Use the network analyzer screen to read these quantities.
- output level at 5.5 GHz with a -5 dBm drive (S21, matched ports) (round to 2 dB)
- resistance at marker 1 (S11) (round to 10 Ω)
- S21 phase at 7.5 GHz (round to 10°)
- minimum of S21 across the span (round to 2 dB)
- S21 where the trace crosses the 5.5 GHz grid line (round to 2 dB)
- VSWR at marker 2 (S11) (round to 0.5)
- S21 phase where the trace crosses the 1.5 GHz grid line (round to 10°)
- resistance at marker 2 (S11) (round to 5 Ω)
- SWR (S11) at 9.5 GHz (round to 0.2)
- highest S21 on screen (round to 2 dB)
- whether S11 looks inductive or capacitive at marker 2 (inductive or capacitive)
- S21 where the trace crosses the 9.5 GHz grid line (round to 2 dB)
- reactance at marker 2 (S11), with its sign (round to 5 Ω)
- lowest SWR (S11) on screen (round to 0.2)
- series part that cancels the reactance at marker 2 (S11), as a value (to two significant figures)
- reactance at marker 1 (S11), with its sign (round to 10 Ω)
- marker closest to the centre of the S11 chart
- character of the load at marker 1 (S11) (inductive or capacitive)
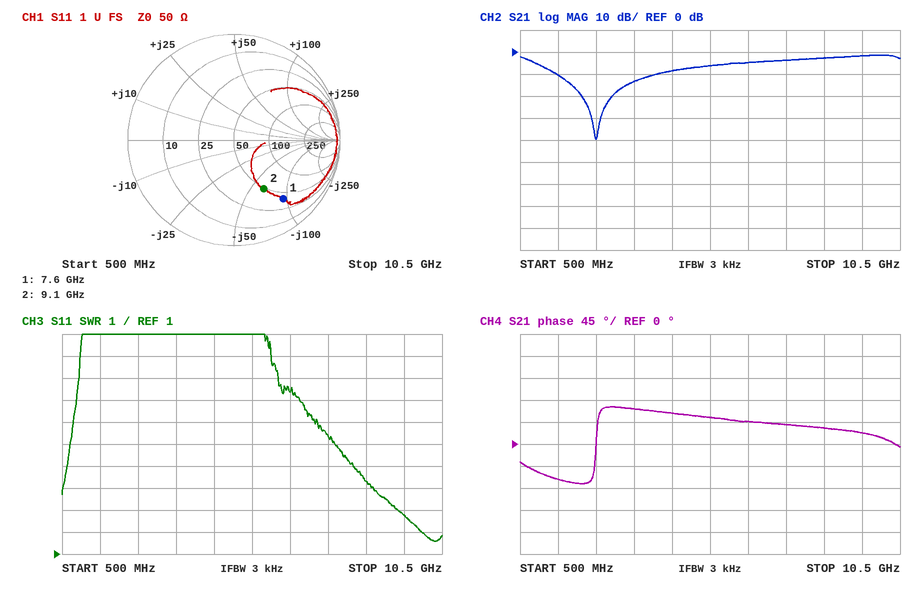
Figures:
-12 dBm
40 Ω
40°
-40 dB
-6 dB
3.5
-70°
50 Ω
2.8
-2 dB
capacitive
-2 dB
-65 Ω
1.6
1.1 nH
-90 Ω
marker 2
capacitive
